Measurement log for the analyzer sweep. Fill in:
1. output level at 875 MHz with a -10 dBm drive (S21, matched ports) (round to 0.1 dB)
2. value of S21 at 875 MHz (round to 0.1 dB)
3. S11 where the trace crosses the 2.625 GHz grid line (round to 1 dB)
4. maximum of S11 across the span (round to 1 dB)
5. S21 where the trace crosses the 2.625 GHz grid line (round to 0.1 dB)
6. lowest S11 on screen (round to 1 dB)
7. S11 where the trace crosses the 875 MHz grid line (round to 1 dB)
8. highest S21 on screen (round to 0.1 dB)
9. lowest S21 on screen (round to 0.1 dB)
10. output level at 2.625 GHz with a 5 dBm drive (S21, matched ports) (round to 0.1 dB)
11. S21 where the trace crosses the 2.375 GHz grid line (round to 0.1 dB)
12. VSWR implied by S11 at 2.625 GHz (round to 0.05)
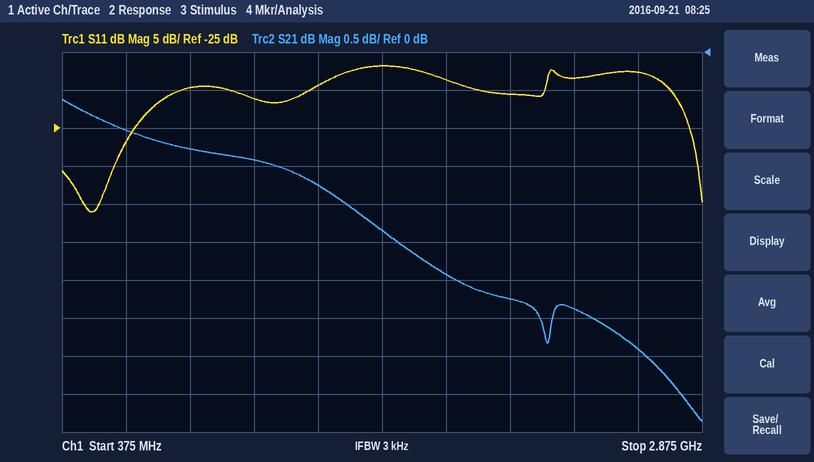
-11.3 dBm
-1.3 dB
-18 dB
-17 dB
-3.9 dB
-36 dB
-20 dB
-0.6 dB
-4.9 dB
1.1 dBm
-3.4 dB
1.30
